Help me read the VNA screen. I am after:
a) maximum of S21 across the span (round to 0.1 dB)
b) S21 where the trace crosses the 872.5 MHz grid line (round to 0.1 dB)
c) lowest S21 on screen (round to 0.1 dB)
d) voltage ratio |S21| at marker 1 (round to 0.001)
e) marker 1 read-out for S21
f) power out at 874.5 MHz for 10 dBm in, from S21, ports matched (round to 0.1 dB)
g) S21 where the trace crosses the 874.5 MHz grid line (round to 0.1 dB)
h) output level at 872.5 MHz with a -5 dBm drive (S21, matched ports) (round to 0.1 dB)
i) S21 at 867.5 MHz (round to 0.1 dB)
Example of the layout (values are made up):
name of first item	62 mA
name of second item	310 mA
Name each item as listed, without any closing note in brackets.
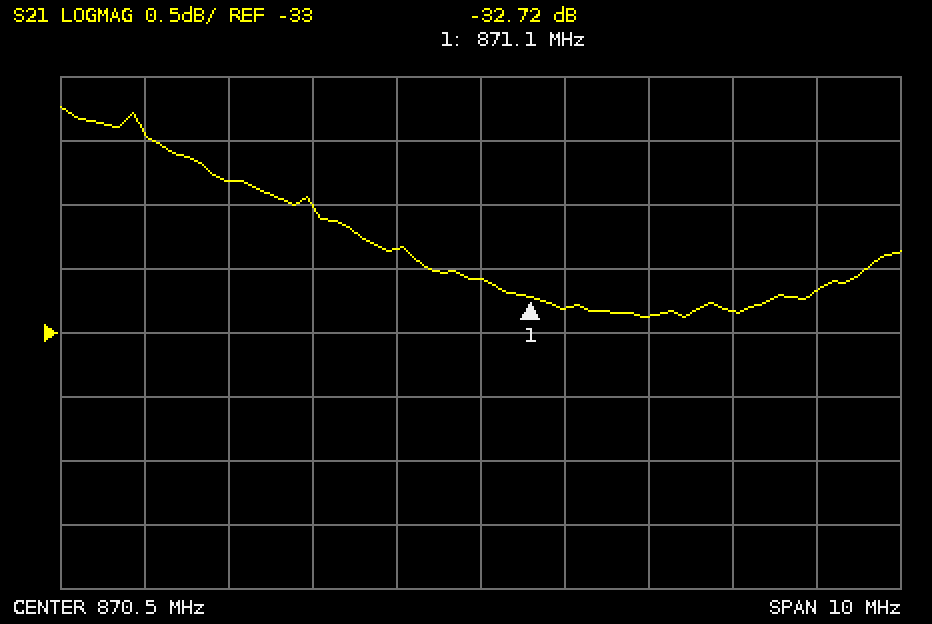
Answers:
maximum of S21 across the span	-31.2 dB
S21 where the trace crosses the 872.5 MHz grid line	-32.9 dB
lowest S21 on screen	-32.9 dB
voltage ratio |S21| at marker 1	0.023
marker 1 read-out for S21	-32.72 dB
power out at 874.5 MHz for 10 dBm in, from S21, ports matched	-22.7 dBm
S21 where the trace crosses the 874.5 MHz grid line	-32.7 dB
output level at 872.5 MHz with a -5 dBm drive (S21, matched ports)	-37.9 dBm
S21 at 867.5 MHz	-31.8 dB
